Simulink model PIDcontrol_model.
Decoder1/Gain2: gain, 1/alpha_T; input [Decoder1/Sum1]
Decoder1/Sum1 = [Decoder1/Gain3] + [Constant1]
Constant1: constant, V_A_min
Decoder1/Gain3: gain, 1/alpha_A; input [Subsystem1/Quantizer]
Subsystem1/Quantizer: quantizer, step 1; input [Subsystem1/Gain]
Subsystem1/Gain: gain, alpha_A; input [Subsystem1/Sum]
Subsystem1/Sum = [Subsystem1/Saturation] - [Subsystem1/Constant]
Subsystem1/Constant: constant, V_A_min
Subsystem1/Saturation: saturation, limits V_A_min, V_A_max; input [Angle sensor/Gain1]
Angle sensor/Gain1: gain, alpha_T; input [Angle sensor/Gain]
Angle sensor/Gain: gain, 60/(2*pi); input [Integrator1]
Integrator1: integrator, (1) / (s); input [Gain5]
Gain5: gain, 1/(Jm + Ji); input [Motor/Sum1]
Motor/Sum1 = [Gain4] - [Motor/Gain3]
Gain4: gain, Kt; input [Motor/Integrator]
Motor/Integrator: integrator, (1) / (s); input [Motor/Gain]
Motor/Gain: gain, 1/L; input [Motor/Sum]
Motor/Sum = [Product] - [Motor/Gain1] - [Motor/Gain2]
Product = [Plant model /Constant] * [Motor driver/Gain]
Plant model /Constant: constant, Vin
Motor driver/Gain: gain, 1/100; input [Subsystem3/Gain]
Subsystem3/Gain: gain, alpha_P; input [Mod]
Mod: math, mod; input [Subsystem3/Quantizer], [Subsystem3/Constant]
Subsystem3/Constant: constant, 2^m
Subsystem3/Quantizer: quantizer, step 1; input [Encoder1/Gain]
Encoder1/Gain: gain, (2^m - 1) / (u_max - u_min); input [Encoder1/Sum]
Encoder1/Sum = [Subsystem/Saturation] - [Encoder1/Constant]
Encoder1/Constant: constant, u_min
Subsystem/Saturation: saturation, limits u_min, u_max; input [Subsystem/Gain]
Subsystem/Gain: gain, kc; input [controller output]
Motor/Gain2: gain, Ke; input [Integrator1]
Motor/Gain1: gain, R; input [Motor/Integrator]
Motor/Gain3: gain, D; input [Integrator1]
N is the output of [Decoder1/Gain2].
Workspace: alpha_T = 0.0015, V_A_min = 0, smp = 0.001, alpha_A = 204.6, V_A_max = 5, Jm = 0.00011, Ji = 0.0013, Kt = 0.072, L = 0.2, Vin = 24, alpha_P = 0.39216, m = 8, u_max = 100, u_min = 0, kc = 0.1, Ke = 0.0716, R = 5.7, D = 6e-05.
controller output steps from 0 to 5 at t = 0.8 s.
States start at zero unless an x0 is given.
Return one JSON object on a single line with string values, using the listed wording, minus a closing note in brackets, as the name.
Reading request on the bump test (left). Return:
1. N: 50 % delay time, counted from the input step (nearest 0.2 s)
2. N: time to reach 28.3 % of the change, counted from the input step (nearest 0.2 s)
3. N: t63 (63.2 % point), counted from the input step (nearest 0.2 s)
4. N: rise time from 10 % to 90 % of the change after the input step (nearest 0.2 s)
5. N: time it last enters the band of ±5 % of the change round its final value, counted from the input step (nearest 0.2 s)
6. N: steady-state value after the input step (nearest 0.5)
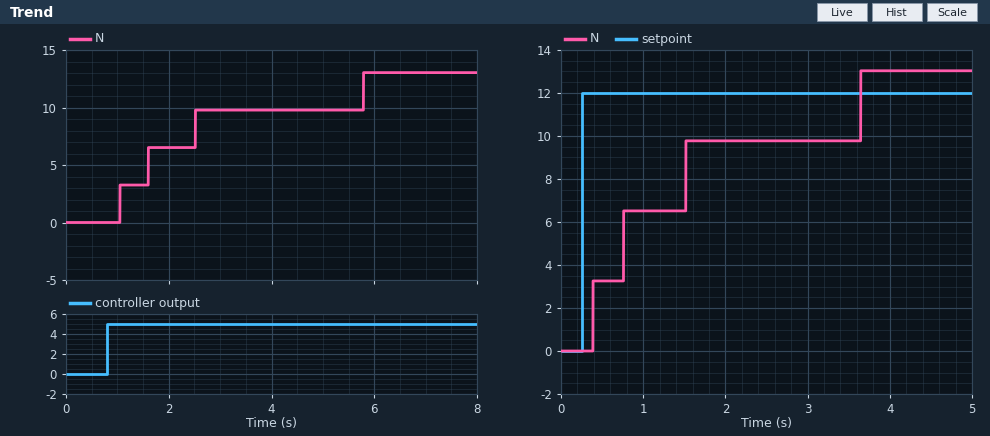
{"N: 50 % delay time, counted from the input step": "0.8 s", "N: time to reach 28.3 % of the change, counted from the input step": "0.8 s", "N: t63 (63.2 % point), counted from the input step": "1.8 s", "N: rise time from 10 % to 90 % of the change after the input step": "4.8 s", "N: time it last enters the band of ±5 % of the change round its final value, counted from the input step": "5.0 s", "N: steady-state value after the input step": "13.0"}
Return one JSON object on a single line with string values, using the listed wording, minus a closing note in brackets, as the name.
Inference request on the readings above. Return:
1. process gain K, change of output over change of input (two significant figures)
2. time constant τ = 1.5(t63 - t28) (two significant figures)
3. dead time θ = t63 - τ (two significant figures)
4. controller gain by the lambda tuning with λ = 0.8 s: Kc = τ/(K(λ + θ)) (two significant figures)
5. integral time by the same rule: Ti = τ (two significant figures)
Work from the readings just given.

{"process gain K, change of output over change of input": "2.6", "time constant τ = 1.5(t63 - t28)": "1.5 s", "dead time θ = t63 - τ": "0.30 s", "controller gain by the lambda tuning with λ = 0.8 s: Kc = τ/(K(λ + θ))": "0.52", "integral time by the same rule: Ti = τ": "1.5 s"}
